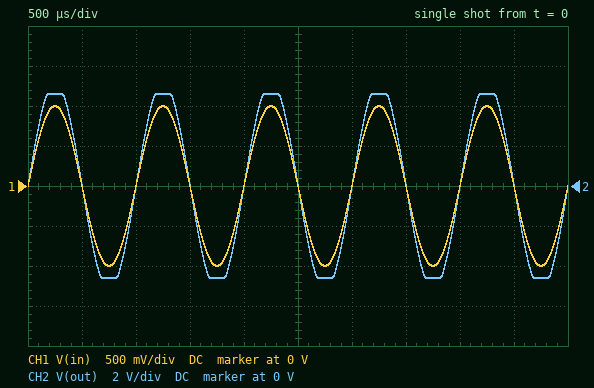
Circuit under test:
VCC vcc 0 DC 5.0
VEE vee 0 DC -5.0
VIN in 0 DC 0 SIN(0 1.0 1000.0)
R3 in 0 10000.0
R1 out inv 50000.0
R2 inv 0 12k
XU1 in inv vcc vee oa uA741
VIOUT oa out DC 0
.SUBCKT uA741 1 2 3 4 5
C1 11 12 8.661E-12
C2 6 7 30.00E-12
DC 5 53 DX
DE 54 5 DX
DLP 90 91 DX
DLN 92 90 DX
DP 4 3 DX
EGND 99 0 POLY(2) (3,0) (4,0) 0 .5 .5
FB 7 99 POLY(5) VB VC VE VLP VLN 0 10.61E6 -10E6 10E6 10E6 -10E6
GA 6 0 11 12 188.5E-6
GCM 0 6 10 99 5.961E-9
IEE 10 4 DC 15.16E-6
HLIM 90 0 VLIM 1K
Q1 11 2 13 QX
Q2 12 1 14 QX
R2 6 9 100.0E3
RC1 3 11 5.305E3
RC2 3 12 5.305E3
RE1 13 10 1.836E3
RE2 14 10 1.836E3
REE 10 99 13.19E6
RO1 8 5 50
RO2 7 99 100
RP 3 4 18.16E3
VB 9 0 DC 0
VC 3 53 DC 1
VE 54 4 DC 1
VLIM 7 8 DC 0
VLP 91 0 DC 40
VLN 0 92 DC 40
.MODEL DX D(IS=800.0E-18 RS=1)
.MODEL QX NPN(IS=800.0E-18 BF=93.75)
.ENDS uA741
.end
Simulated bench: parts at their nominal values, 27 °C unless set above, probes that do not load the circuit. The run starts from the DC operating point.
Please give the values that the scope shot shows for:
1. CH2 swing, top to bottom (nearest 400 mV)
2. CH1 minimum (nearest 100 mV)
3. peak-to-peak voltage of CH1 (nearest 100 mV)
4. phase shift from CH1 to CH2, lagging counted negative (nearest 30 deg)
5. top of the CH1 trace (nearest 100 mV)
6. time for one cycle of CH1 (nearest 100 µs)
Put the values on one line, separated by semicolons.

9.2 V; -1.0 V; 2.0 V; 0 deg; 1.0 V; 1.0 ms
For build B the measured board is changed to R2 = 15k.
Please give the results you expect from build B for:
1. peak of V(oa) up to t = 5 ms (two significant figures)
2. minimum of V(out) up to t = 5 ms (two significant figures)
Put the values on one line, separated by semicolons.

4.3 V; -4.3 V
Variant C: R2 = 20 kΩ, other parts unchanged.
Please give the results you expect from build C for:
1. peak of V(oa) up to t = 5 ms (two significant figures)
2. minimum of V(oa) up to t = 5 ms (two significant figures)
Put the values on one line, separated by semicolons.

3.5 V; -3.5 V
